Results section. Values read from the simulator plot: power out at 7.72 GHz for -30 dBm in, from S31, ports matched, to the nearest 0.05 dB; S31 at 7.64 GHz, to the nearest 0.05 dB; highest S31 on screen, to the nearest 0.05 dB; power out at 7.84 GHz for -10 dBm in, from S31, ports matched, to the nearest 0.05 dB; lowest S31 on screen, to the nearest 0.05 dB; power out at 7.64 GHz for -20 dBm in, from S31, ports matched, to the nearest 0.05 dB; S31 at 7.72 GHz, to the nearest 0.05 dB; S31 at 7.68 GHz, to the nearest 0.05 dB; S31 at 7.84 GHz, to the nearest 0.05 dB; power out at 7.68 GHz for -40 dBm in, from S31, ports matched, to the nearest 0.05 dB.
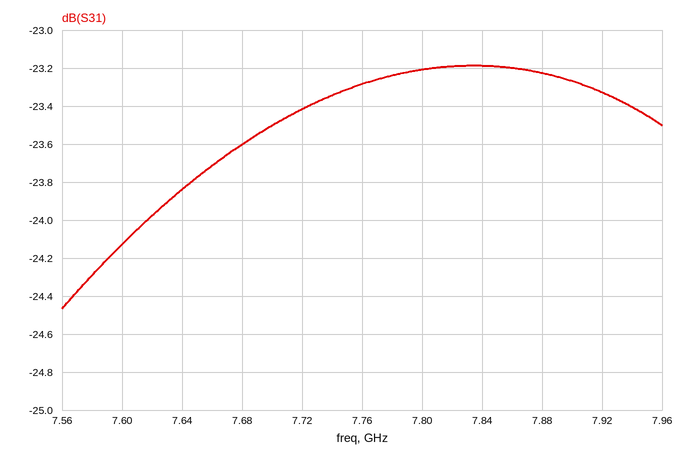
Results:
-53.40 dBm
-23.85 dB
-23.20 dB
-33.20 dBm
-24.45 dB
-43.85 dBm
-23.40 dB
-23.60 dB
-23.20 dB
-63.60 dBm
